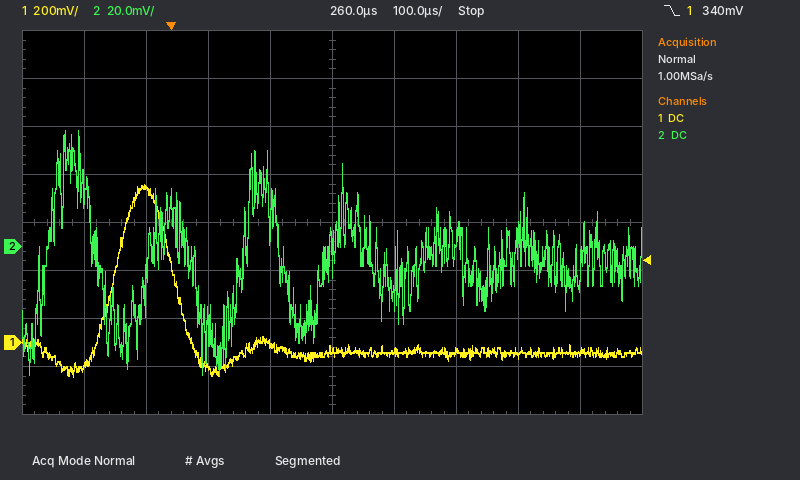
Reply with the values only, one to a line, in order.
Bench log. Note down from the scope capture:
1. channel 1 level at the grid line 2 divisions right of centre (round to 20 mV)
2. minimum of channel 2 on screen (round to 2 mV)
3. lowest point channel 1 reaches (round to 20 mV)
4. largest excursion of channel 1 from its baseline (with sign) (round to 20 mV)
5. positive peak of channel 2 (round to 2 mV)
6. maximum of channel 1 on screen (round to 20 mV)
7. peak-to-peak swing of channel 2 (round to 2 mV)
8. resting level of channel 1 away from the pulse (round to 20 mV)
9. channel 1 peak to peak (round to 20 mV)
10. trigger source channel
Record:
-40 mV
-54 mV
-140 mV
+700 mV
48 mV
660 mV
102 mV
-40 mV
800 mV
channel 1
